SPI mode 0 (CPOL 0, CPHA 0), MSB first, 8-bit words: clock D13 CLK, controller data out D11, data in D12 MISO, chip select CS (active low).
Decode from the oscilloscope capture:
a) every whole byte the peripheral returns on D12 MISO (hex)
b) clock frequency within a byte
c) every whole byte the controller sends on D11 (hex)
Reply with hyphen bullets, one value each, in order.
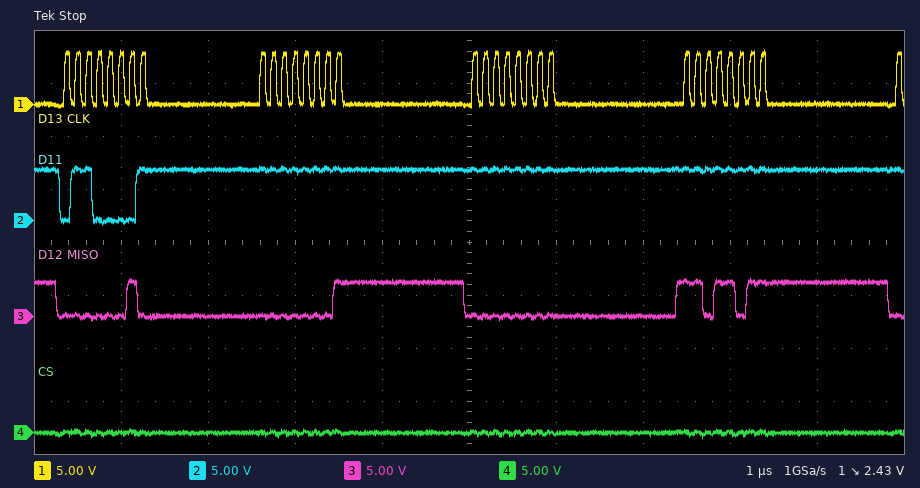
- 0x02 0x01 0x00 0xDB
- 8 MHz
- 0x61 0xFF 0xFF 0xFF
